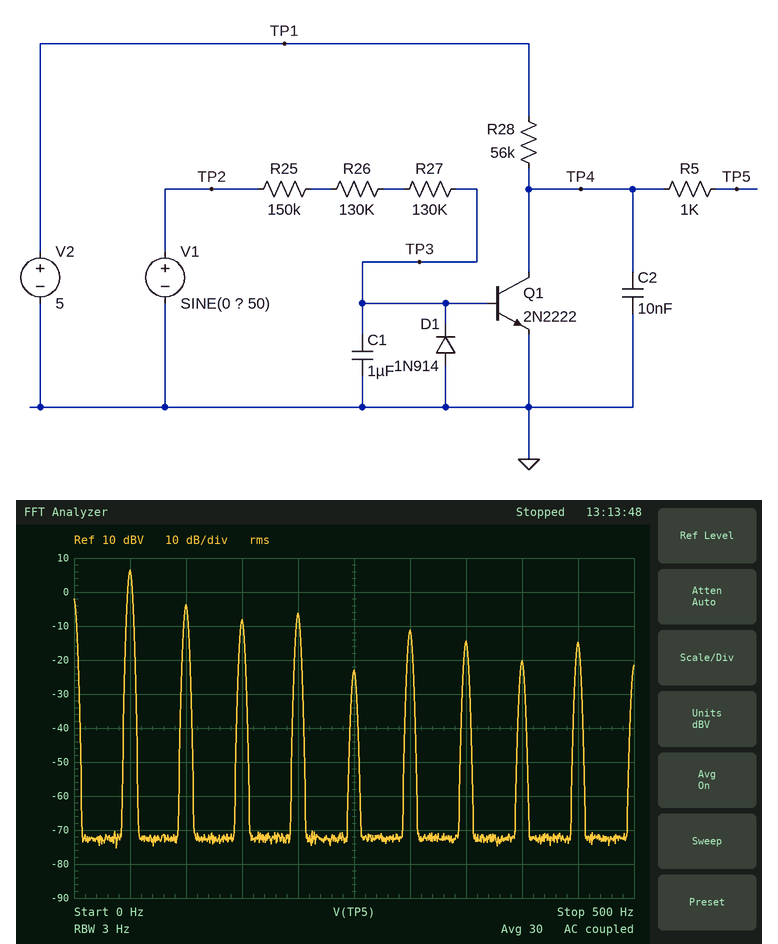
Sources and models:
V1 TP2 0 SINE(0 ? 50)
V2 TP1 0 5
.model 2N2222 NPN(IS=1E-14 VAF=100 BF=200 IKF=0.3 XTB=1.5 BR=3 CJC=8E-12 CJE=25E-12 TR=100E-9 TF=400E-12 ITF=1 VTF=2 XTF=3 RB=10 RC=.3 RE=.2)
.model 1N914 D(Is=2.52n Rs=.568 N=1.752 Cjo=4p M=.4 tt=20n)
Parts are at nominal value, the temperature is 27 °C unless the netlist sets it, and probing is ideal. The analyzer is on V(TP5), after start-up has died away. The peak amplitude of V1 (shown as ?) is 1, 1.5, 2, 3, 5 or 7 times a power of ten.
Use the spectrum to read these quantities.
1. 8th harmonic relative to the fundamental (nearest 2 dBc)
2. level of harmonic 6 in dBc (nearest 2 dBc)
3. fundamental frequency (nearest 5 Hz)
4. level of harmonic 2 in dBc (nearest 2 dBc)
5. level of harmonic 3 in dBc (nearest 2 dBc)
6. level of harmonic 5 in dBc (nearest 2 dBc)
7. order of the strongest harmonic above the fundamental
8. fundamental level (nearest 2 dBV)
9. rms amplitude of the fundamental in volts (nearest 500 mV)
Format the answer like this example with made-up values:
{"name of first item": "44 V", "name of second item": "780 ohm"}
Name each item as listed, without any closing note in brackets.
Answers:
{"8th harmonic relative to the fundamental": "-26 dBc", "level of harmonic 6 in dBc": "-18 dBc", "fundamental frequency": "50 Hz", "level of harmonic 2 in dBc": "-10 dBc", "level of harmonic 3 in dBc": "-14 dBc", "level of harmonic 5 in dBc": "-30 dBc", "order of the strongest harmonic above the fundamental": "2", "fundamental level": "6 dBV", "rms amplitude of the fundamental in volts": "2.0 V"}
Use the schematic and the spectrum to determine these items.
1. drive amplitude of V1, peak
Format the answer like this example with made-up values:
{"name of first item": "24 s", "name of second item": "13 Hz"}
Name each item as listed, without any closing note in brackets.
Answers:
{"drive amplitude of V1, peak": "300 V"}
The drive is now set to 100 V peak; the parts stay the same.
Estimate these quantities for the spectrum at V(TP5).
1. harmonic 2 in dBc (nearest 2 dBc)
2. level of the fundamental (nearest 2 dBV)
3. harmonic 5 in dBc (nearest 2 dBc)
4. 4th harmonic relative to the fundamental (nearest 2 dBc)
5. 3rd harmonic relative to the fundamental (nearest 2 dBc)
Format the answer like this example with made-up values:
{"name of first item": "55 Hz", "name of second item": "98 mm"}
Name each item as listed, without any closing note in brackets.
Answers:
{"harmonic 2 in dBc": "-4 dBc", "level of the fundamental": "4 dBV", "harmonic 5 in dBc": "-14 dBc", "4th harmonic relative to the fundamental": "-22 dBc", "3rd harmonic relative to the fundamental": "-12 dBc"}
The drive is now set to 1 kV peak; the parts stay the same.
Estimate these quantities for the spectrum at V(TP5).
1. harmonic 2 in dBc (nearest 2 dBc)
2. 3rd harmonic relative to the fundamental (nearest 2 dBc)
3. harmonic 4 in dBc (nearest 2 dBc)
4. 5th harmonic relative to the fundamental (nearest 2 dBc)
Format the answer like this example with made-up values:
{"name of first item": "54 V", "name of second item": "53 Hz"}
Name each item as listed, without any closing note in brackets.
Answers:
{"harmonic 2 in dBc": "-18 dBc", "3rd harmonic relative to the fundamental": "-10 dBc", "harmonic 4 in dBc": "-18 dBc", "5th harmonic relative to the fundamental": "-18 dBc"}
